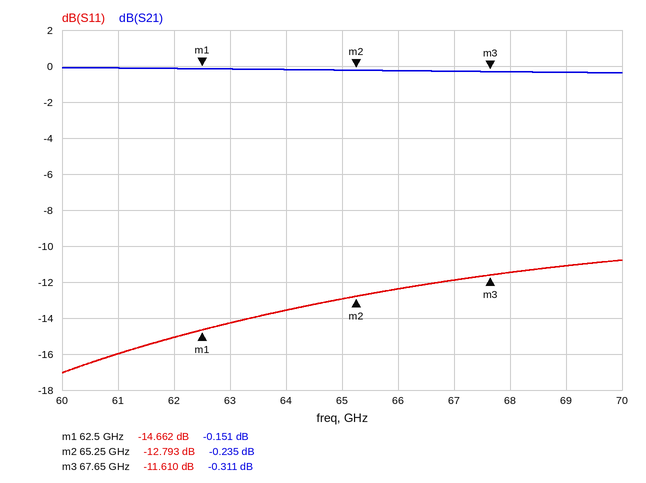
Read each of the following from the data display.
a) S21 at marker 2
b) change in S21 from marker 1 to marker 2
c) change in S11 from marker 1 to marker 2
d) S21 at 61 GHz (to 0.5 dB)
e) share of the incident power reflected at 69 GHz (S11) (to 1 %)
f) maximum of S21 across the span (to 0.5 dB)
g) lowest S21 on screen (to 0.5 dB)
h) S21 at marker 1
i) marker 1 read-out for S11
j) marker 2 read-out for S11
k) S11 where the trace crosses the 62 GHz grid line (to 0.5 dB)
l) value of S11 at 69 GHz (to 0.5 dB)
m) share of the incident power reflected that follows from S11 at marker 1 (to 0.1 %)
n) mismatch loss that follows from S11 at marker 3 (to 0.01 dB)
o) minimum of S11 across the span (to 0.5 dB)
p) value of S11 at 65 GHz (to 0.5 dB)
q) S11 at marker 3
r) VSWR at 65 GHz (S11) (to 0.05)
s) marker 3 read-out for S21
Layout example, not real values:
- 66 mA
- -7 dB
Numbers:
- -0.235 dB
- -0.084 dB
- 1.869 dB
- 0.0 dB
- 8 %
- 0.0 dB
- -0.5 dB
- -0.151 dB
- -14.662 dB
- -12.793 dB
- -15.0 dB
- -11.0 dB
- 3.4 %
- 0.31 dB
- -17.0 dB
- -13.0 dB
- -11.610 dB
- 1.60
- -0.311 dB
